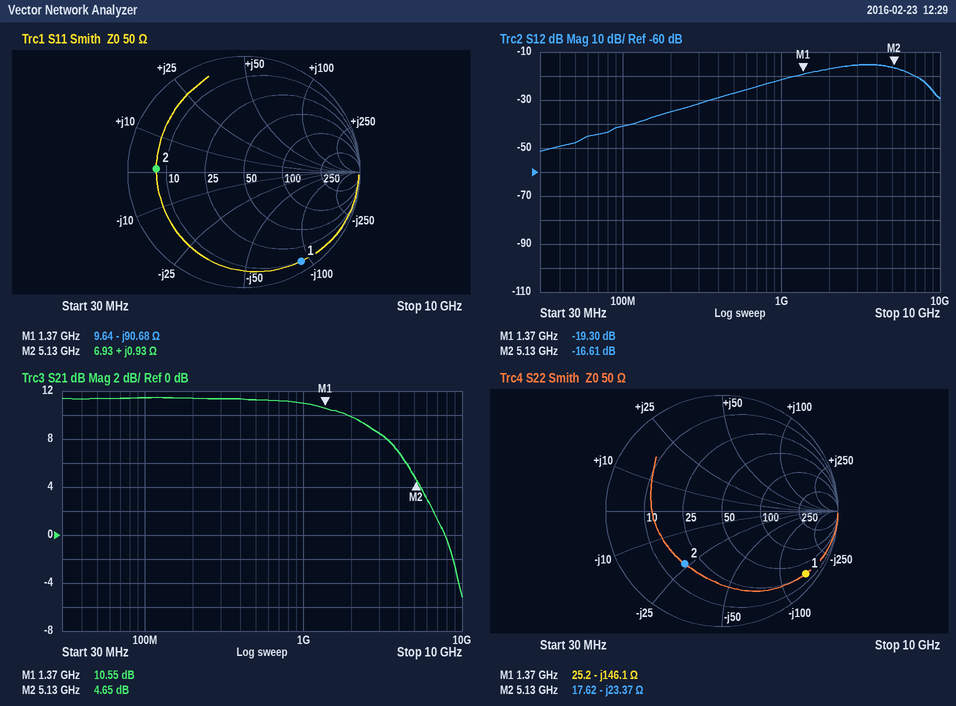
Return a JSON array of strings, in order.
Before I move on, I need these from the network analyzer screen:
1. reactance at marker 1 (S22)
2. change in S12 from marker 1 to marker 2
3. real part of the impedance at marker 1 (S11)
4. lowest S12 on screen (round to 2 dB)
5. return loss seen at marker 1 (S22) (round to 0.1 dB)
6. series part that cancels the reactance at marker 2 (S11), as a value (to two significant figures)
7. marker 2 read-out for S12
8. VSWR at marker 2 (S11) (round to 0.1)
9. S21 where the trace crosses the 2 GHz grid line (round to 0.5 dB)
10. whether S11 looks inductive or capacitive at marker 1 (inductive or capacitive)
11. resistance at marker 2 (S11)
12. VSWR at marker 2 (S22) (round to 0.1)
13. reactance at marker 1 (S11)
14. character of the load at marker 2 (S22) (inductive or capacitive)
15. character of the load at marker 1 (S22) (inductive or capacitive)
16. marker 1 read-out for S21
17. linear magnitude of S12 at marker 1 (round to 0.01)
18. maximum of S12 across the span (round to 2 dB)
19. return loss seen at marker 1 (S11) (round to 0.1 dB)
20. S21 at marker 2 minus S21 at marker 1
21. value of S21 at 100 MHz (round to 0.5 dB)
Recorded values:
["-146.1 Ω", "2.69 dB", "9.64 Ω", "-52 dB", "0.9 dB", "33 pF", "-16.61 dB", "7.2", "10.0 dB", "capacitive", "6.93 Ω", "3.5", "-90.68 Ω", "capacitive", "capacitive", "10.55 dB", "0.11", "-16 dB", "0.8 dB", "-5.90 dB", "11.5 dB"]
